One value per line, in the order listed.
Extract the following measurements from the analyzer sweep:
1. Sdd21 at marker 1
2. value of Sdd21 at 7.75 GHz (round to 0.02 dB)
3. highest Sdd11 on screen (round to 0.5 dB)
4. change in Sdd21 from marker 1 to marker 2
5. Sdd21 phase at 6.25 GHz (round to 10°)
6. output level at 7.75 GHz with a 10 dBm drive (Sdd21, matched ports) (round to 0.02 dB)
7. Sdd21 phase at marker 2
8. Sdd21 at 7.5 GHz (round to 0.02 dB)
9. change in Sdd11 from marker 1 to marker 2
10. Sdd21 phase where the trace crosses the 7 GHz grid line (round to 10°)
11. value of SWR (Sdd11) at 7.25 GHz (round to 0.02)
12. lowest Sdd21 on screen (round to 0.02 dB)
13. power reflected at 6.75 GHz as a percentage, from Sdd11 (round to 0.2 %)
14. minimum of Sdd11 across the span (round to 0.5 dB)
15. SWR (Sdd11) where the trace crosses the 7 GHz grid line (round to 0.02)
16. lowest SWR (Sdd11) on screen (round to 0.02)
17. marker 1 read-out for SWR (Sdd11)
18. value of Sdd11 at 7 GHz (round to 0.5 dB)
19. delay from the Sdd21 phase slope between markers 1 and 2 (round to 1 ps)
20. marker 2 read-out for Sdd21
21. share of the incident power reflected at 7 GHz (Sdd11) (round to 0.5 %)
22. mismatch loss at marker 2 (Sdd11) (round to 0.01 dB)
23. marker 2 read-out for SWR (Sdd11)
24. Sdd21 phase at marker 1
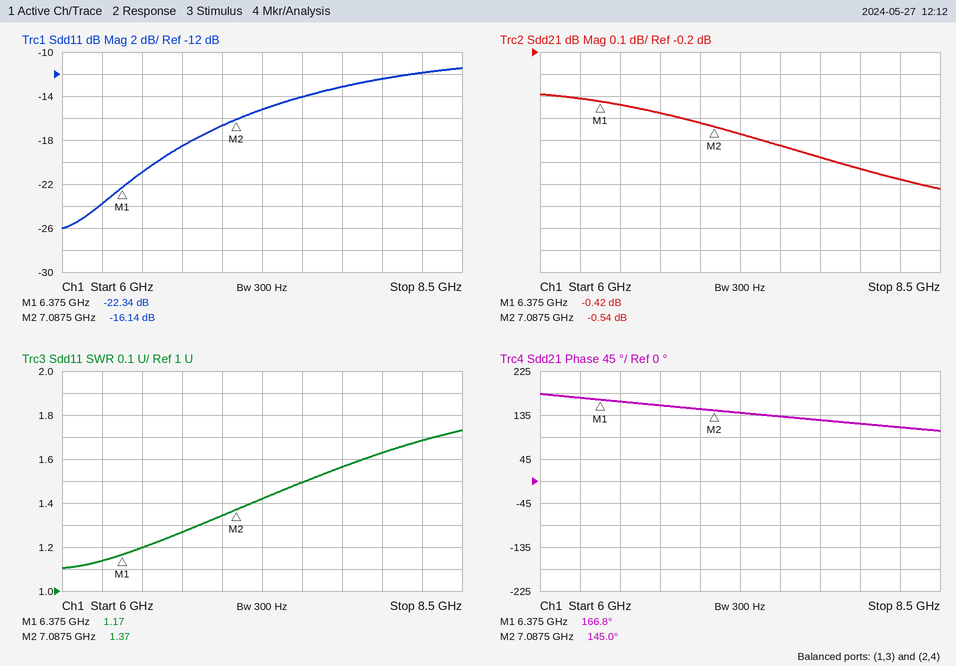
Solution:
-0.42 dB
-0.68 dB
-11.5 dB
-0.12 dB
170°
9.32 dBm
145.0°
-0.62 dB
6.20 dB
150°
1.42
-0.82 dB
1.4 %
-26.0 dB
1.34
1.10
1.17
-16.5 dB
85 ps
-0.54 dB
2.0 %
0.11 dB
1.37
166.8°
